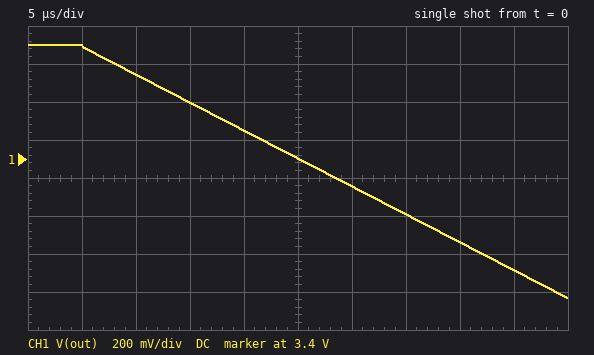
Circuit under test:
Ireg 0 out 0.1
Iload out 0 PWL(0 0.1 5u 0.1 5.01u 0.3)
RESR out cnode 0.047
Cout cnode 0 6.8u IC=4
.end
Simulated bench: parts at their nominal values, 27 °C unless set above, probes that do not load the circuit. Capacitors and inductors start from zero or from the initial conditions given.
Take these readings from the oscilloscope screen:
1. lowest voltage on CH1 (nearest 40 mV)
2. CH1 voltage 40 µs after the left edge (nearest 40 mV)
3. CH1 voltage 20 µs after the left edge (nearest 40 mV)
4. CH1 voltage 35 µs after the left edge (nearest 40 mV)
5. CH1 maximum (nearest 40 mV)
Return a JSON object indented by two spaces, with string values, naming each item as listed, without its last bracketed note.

{
  "lowest voltage on CH1": "2.68 V",
  "CH1 voltage 40 µs after the left edge": "2.96 V",
  "CH1 voltage 20 µs after the left edge": "3.56 V",
  "CH1 voltage 35 µs after the left edge": "3.12 V",
  "CH1 maximum": "4.00 V"
}
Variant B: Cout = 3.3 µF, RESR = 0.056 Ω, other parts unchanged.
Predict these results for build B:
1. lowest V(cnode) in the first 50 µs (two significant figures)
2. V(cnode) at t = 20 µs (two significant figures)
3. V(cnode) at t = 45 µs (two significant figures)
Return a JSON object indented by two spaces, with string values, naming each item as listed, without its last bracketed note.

{
  "lowest V(cnode) in the first 50 µs": "1.3 V",
  "V(cnode) at t = 20 µs": "3.1 V",
  "V(cnode) at t = 45 µs": "1.6 V"
}
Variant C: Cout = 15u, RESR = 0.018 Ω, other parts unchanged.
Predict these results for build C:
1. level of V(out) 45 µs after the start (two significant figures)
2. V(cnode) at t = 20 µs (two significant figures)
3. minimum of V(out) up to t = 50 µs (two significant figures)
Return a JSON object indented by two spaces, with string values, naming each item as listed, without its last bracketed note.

{
  "level of V(out) 45 µs after the start": "3.5 V",
  "V(cnode) at t = 20 µs": "3.8 V",
  "minimum of V(out) up to t = 50 µs": "3.4 V"
}
